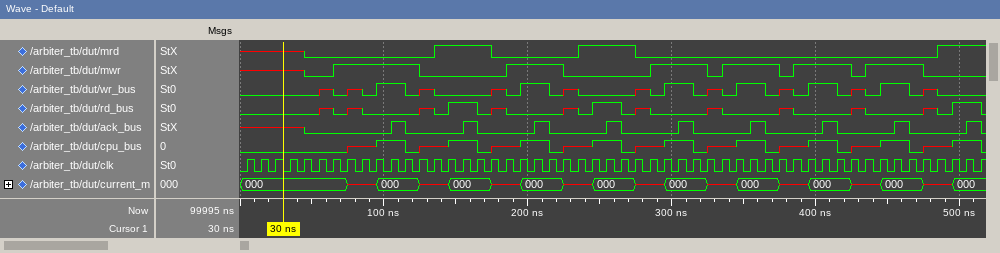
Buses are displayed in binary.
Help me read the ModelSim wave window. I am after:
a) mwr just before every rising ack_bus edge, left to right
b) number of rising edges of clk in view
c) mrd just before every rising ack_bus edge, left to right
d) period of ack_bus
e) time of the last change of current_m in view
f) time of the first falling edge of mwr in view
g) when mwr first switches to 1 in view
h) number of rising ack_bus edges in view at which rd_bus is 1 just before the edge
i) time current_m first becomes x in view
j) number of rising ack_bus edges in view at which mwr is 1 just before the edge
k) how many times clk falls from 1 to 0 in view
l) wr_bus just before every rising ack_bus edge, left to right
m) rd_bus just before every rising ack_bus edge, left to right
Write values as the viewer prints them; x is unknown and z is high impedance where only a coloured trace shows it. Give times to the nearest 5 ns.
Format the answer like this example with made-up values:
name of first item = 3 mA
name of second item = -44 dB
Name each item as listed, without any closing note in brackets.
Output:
mwr just before every rising ack_bus edge, left to right = 1 0 1 0 1 1 1 1 0
number of rising edges of clk in view = 52
mrd just before every rising ack_bus edge, left to right = 0 1 0 1 0 0 0 0 1
period of ack_bus = 50 ns
time of the last change of current_m in view = 495 ns
time of the first falling edge of mwr in view = 125 ns
when mwr first switches to 1 in view = 65 ns
number of rising ack_bus edges in view at which rd_bus is 1 just before the edge = 3
time current_m first becomes x in view = 75 ns
number of rising ack_bus edges in view at which mwr is 1 just before the edge = 6
how many times clk falls from 1 to 0 in view = 51
wr_bus just before every rising ack_bus edge, left to right = 1 0 1 0 1 1 1 1 0
rd_bus just before every rising ack_bus edge, left to right = 0 1 0 1 0 0 0 0 1
